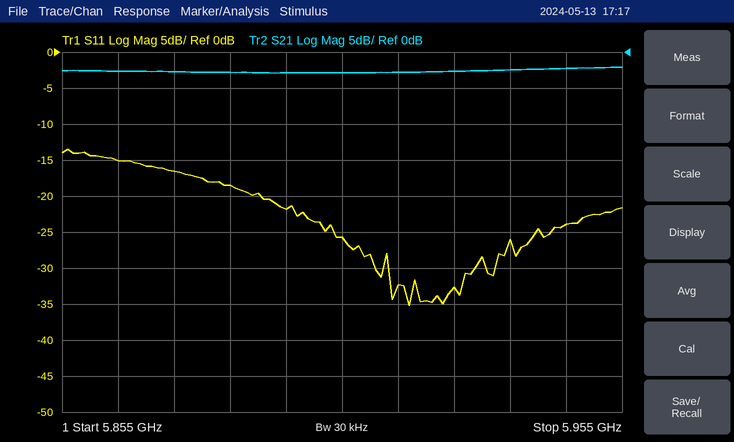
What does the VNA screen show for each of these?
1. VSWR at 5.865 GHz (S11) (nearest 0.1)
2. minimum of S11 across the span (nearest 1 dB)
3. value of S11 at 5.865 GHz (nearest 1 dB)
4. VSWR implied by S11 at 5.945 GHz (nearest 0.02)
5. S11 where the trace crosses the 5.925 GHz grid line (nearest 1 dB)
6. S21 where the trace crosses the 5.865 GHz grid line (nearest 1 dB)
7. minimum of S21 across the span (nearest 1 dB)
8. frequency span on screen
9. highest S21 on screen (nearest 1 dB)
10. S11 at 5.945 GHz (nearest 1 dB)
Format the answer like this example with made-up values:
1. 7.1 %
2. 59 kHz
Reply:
1. 1.4
2. -35 dB
3. -15 dB
4. 1.14
5. -33 dB
6. -3 dB
7. -3 dB
8. 100 MHz
9. -2 dB
10. -24 dB
